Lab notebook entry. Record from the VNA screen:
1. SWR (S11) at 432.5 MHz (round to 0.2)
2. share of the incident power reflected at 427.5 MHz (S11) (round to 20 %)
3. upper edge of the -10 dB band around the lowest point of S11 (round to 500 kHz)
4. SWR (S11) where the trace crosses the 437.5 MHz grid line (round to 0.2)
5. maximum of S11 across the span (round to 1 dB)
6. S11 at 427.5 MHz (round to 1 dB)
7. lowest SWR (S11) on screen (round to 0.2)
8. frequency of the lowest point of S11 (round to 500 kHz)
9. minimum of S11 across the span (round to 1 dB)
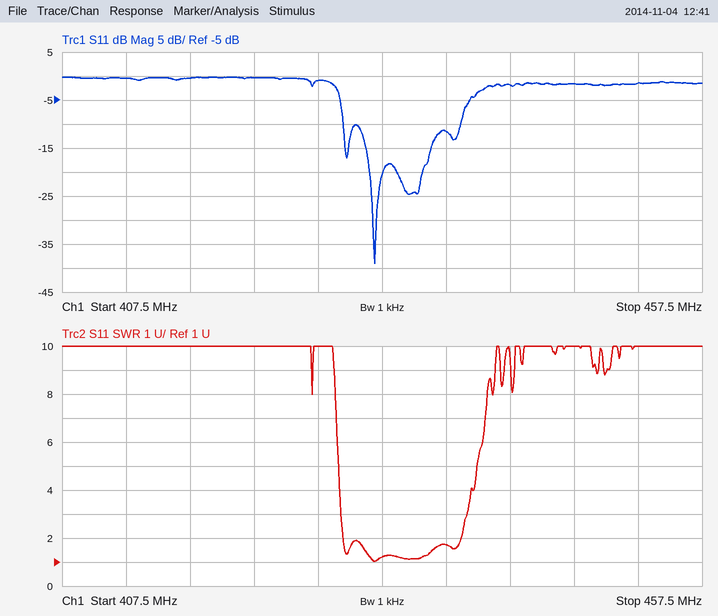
1.2
80 %
438.5 MHz
1.8
0 dB
-1 dB
1.0
432.0 MHz
-39 dB
